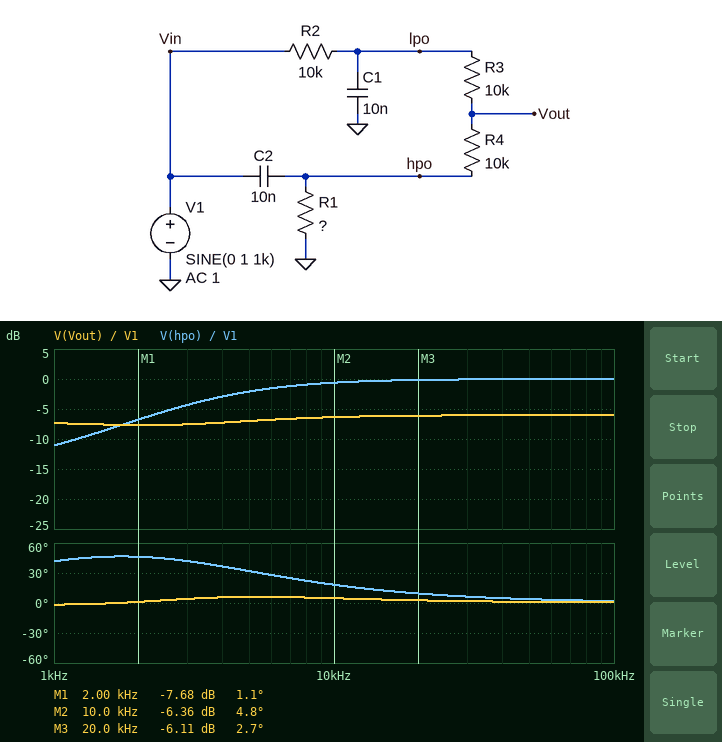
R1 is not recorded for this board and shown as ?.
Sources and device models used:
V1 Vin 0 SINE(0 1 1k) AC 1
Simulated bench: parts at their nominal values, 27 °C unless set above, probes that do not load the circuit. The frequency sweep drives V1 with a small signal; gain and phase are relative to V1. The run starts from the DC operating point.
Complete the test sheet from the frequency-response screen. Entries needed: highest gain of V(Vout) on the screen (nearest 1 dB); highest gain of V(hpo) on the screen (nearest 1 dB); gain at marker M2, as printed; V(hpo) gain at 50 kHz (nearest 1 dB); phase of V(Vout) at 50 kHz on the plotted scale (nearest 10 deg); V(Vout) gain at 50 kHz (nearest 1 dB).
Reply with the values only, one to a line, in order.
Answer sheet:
-6 dB
0 dB
-6.36 dB
0 dB
0 deg
-6 dB
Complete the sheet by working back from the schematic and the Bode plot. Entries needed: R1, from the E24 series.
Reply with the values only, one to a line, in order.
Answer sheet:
6.2 kΩ
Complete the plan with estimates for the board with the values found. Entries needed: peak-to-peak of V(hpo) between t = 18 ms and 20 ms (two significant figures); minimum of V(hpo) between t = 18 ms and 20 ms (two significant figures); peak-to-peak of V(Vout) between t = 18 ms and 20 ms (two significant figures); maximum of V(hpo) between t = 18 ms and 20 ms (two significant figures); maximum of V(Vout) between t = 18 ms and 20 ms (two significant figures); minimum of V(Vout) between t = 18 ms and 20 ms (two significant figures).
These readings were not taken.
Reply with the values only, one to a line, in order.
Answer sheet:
560 mV
-280 mV
860 mV
280 mV
430 mV
-430 mV
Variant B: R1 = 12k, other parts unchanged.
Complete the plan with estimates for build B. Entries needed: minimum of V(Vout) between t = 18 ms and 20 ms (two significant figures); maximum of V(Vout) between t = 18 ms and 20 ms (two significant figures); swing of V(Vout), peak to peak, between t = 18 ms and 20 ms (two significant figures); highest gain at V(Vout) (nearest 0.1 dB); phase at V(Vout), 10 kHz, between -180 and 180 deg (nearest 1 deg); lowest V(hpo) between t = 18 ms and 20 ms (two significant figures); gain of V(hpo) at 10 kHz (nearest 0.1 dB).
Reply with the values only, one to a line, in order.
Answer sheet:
-530 mV
530 mV
1.1 V
-5.5 dB
-1 deg
-420 mV
-0.3 dB
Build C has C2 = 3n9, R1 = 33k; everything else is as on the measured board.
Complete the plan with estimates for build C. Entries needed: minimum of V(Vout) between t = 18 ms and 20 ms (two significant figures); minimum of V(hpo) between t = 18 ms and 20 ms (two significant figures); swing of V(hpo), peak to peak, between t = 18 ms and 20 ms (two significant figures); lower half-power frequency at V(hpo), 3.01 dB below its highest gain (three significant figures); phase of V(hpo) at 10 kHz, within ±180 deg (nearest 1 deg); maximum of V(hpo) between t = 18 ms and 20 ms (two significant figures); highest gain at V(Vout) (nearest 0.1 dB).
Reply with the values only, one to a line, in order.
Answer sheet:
-580 mV
-430 mV
850 mV
4.70 kHz
17 deg
430 mV
-3.3 dB
